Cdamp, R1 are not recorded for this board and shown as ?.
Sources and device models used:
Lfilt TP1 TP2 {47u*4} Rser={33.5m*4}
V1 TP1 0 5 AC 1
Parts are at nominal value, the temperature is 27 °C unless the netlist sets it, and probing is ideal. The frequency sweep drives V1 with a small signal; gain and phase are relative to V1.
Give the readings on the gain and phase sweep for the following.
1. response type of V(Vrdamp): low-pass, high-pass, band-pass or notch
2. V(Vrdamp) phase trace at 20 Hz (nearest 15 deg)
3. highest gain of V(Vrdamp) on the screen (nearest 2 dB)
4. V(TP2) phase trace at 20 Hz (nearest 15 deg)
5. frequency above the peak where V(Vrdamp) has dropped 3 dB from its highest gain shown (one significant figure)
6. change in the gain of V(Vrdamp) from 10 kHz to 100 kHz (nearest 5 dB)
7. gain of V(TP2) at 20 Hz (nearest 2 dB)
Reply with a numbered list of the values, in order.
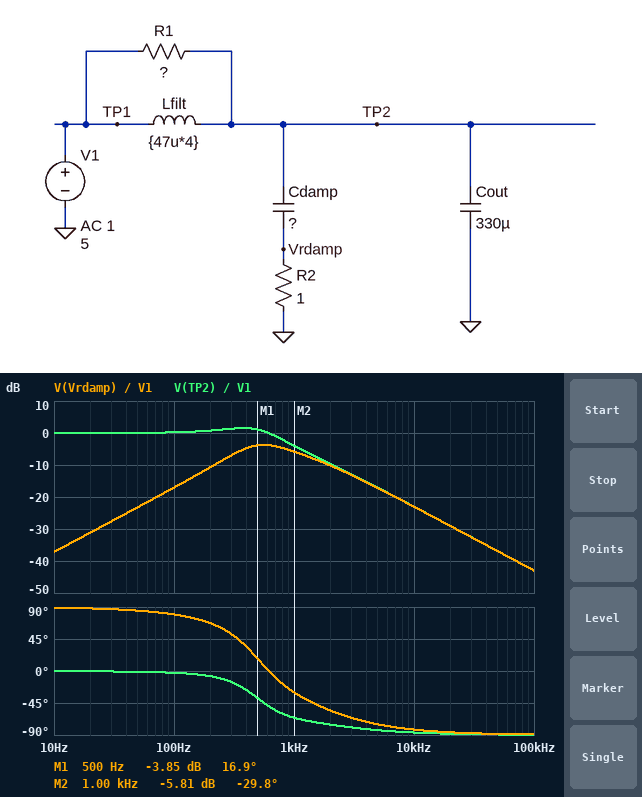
1. band-pass
2. 90 deg
3. -4 dB
4. 0 deg
5. 1 kHz
6. -20 dB
7. 0 dB
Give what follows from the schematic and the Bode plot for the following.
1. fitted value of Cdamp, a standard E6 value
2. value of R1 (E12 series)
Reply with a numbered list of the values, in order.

1. 220 µF
2. 0.68 Ω
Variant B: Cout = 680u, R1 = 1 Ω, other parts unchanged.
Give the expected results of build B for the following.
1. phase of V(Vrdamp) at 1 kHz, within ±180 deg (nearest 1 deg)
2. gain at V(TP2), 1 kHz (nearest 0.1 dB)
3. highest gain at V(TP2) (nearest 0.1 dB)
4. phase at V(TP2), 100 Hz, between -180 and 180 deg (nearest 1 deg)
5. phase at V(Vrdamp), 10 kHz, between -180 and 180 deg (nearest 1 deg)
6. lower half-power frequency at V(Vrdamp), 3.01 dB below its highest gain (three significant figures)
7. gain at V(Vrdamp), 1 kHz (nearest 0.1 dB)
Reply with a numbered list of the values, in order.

1. -67 deg
2. -9.9 dB
3. 3.2 dB
4. -4 deg
5. -88 deg
6. 273 Hz
7. -11.7 dB
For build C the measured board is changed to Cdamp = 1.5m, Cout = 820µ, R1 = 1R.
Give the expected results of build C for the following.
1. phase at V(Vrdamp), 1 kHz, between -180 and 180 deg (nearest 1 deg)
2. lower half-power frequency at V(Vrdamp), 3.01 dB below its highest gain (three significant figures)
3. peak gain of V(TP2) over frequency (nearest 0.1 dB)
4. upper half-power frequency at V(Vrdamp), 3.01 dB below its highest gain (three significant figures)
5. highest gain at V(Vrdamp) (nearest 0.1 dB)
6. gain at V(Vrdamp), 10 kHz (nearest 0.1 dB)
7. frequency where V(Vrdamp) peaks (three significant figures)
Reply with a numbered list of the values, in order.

1. -96 deg
2. 107 Hz
3. 0.7 dB
4. 539 Hz
5. 0.2 dB
6. -34.2 dB
7. 309 Hz
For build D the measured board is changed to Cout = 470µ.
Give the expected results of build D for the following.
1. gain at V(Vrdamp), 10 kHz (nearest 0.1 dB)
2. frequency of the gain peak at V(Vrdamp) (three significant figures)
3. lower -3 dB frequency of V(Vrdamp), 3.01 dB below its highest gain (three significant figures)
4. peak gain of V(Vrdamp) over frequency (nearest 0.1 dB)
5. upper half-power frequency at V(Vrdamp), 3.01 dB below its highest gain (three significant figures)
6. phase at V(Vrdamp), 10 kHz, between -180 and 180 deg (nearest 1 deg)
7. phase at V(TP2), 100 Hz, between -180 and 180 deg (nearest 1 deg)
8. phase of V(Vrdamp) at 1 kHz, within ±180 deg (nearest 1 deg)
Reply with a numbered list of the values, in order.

1. -26.1 dB
2. 495 Hz
3. 290 Hz
4. -3.9 dB
5. 923 Hz
6. -84 deg
7. -3 deg
8. -42 deg
